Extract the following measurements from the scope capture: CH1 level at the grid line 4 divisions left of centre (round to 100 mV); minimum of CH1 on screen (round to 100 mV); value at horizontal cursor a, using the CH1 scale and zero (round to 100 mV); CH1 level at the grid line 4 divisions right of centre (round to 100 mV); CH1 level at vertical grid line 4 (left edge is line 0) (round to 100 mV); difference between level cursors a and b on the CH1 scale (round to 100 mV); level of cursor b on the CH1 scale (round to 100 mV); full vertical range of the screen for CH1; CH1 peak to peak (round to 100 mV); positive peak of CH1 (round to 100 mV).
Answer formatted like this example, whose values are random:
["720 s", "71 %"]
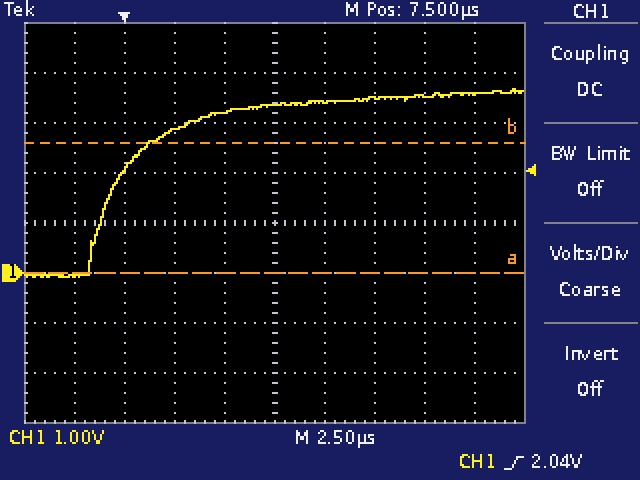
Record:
["-100 mV", "-100 mV", "0.0 V", "3.6 V", "3.2 V", "2.6 V", "2.6 V", "8 V", "3.8 V", "3.7 V"]
